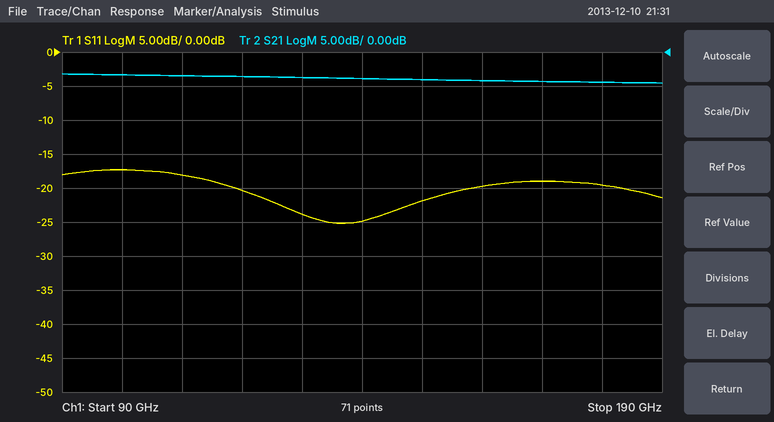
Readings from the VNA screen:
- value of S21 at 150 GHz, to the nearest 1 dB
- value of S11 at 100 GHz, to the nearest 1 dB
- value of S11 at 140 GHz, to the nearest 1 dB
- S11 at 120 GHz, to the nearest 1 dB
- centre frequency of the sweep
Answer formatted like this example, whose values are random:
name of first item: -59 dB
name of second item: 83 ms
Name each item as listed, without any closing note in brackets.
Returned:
value of S21 at 150 GHz, to the nearest 1 dB: -4 dB
value of S11 at 100 GHz, to the nearest 1 dB: -17 dB
value of S11 at 140 GHz, to the nearest 1 dB: -25 dB
S11 at 120 GHz, to the nearest 1 dB: -20 dB
centre frequency of the sweep: 140 GHz
